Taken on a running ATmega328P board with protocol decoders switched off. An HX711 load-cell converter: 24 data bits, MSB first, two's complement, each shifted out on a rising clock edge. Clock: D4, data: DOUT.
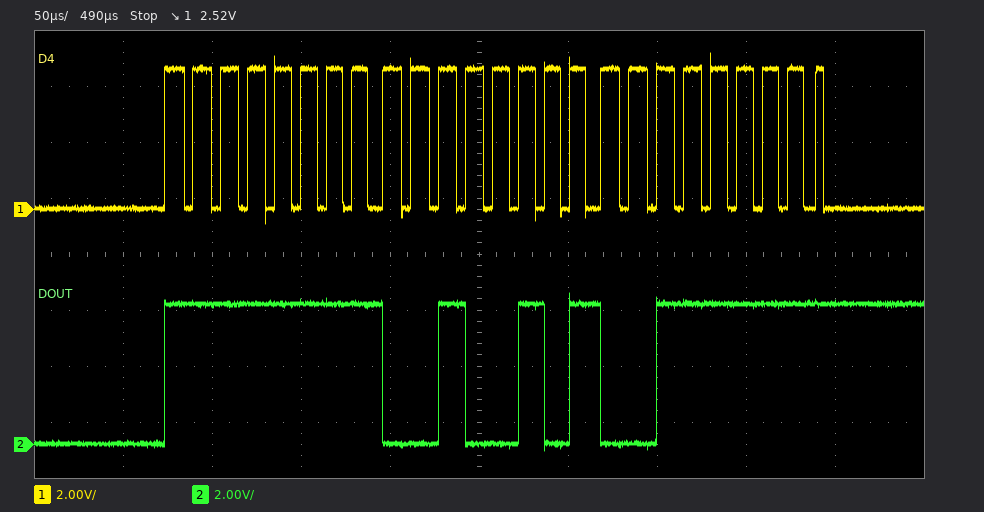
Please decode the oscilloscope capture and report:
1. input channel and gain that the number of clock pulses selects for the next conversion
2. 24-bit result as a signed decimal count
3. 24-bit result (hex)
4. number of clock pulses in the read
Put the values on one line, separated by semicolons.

channel A, gain 128; -56001; 0xFF253F; 25
